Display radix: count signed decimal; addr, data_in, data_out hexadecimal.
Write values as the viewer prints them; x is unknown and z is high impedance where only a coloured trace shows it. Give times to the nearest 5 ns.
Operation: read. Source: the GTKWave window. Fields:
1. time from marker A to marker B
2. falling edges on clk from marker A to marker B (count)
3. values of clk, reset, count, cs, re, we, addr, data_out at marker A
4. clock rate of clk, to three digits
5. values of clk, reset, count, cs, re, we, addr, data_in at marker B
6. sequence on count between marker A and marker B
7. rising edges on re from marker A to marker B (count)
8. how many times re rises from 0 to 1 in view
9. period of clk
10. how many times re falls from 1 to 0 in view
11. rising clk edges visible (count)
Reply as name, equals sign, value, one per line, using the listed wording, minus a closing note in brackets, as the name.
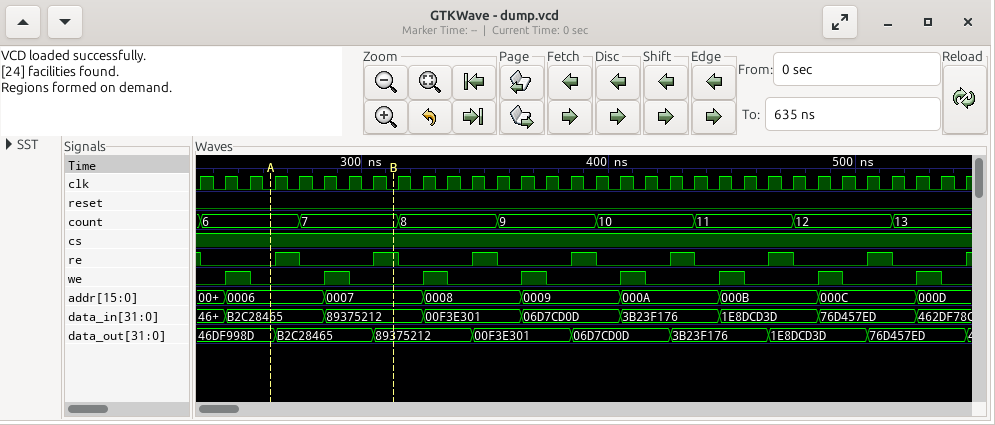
time from marker A to marker B = 50 ns
falling edges on clk from marker A to marker B = 5
values of clk, reset, count, cs, re, we, addr, data_out at marker A = clk=0, reset=0, count=6, cs=1, re=0, we=0, addr=0006, data_out=46DF998D
clock rate of clk, to three digits = 100 MHz
values of clk, reset, count, cs, re, we, addr, data_in at marker B = clk=0, reset=0, count=7, cs=1, re=1, we=0, addr=0007, data_in=89375212
sequence on count between marker A and marker B = 6, 7
rising edges on re from marker A to marker B = 2
how many times re rises from 0 to 1 in view = 8
period of clk = 10 ns
how many times re falls from 1 to 0 in view = 8
rising clk edges visible = 32
